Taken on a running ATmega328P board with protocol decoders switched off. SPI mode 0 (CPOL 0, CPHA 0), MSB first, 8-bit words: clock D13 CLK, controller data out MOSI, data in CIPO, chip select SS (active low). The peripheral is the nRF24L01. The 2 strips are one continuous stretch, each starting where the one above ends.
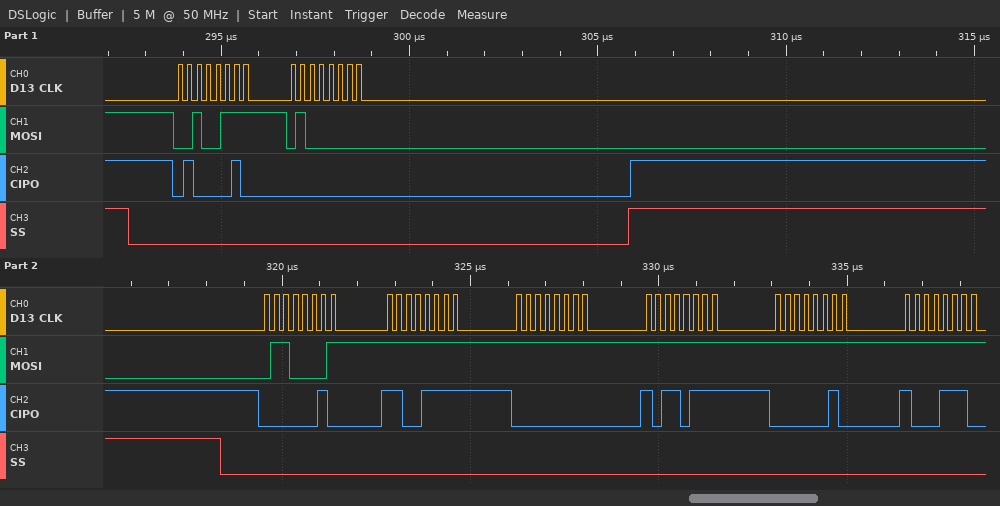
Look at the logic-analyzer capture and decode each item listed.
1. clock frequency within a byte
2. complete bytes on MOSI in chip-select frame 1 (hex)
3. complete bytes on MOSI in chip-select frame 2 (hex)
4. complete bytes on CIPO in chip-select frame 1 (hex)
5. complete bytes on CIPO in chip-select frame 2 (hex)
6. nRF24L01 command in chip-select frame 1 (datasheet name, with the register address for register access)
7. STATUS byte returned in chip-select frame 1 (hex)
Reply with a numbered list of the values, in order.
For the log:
1. 4 MHz
2. 0x27 0x40
3. 0x61 0xFF 0xFF 0xFF 0xFF 0xFF
4. 0x42 0x00
5. 0x02 0xCF 0x00 0xB7 0x02 0x8E
6. W_REGISTER 0x07
7. 0x42
